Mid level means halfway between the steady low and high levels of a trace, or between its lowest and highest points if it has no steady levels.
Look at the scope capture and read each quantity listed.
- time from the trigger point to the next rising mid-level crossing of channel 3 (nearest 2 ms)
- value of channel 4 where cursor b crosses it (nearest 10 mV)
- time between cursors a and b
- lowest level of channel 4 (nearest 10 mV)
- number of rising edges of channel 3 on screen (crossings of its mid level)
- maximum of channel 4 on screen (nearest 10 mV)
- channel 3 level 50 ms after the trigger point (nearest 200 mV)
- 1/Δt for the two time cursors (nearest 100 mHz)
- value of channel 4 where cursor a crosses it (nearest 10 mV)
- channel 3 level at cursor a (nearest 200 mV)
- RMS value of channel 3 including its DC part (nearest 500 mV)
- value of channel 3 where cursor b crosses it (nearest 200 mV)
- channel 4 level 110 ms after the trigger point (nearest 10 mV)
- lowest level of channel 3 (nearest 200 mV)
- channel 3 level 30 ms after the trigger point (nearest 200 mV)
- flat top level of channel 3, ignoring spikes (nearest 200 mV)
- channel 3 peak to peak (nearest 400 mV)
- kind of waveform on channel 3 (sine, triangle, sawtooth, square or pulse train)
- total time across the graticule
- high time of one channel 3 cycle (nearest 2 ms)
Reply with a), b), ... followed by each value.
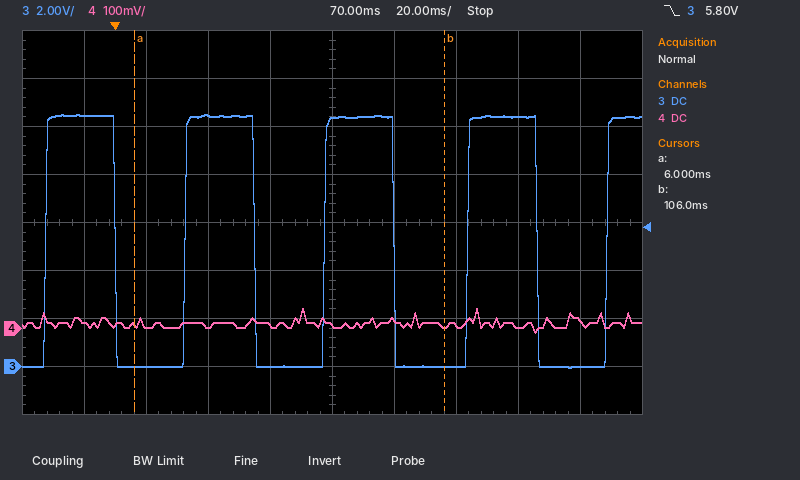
a) 22 ms
b) 0 mV
c) 100 ms
d) -10 mV
e) 5
f) 40 mV
g) 0.0 V
h) 10.0 Hz
i) 10 mV
j) 0.0 V
k) 7.5 V
l) 0.0 V
m) 10 mV
n) 0.0 V
o) 10.4 V
p) 10.4 V
q) 10.4 V
r) square
s) 200 ms
t) 22 ms
